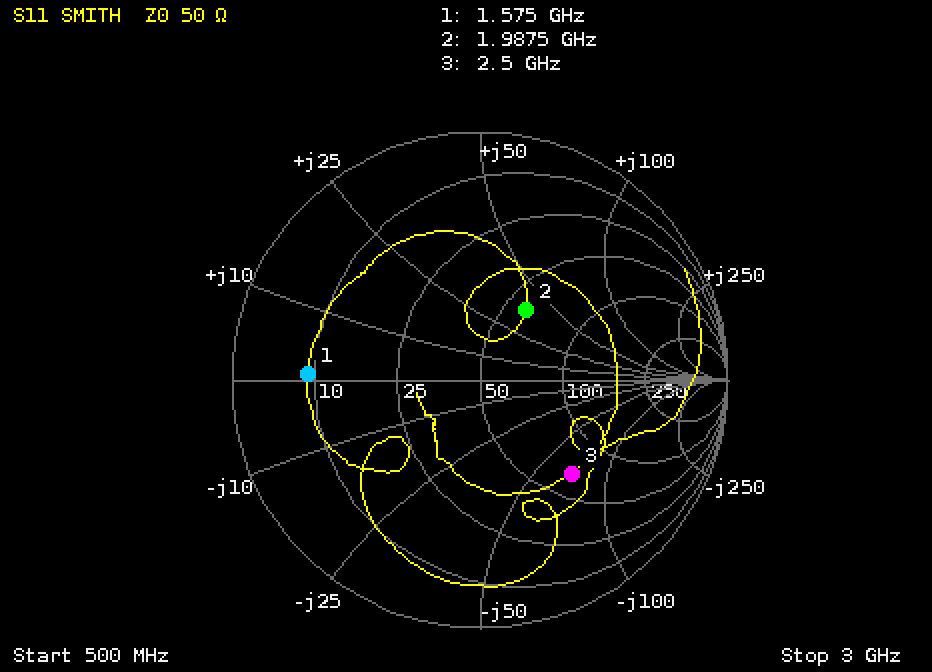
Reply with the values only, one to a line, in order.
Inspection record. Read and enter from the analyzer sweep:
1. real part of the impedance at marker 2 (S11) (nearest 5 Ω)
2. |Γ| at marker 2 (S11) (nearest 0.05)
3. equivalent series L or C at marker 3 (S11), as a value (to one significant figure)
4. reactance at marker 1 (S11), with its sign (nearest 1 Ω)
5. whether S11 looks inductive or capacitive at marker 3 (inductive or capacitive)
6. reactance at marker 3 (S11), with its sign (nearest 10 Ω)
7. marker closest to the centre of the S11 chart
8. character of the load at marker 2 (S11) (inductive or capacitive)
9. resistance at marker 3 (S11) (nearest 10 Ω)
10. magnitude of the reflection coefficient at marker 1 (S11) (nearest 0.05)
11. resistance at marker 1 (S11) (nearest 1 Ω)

60 Ω
0.35
900 fF
+1 Ω
capacitive
-70 Ω
marker 2
inductive
70 Ω
0.70
9 Ω
